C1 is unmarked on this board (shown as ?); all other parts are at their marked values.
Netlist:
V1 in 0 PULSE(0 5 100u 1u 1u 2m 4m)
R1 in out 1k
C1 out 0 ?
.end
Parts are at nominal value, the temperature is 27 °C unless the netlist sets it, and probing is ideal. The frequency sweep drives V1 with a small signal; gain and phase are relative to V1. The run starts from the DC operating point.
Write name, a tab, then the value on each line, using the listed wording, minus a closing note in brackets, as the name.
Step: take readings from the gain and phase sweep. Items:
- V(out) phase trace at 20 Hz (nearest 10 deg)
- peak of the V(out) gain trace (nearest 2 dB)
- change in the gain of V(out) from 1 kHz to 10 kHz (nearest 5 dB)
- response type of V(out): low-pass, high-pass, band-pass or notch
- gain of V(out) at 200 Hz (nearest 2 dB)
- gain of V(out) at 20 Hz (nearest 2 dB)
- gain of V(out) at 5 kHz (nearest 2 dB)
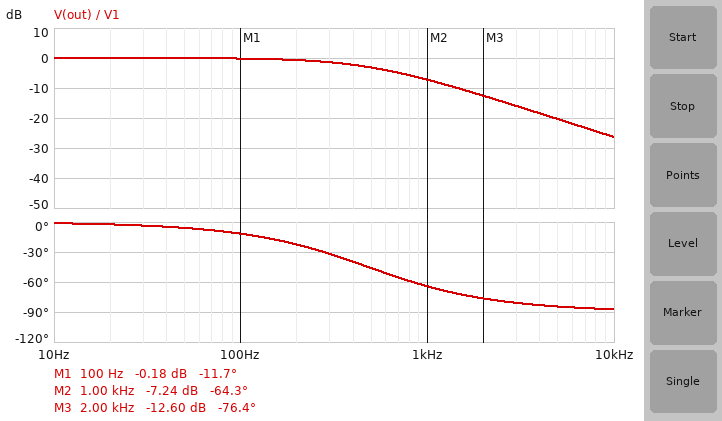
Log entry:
V(out) phase trace at 20 Hz	0 deg
peak of the V(out) gain trace	0 dB
change in the gain of V(out) from 1 kHz to 10 kHz	-20 dB
response type of V(out): low-pass, high-pass, band-pass or notch	low-pass
gain of V(out) at 200 Hz	0 dB
gain of V(out) at 20 Hz	0 dB
gain of V(out) at 5 kHz	-20 dB
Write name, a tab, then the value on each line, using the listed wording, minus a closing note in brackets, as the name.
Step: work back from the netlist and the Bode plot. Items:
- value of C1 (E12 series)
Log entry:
value of C1	330 nF
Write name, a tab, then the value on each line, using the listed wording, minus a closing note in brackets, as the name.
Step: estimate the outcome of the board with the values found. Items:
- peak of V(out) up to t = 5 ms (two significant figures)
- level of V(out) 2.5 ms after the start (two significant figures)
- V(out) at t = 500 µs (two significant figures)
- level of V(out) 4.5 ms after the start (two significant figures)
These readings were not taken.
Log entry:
peak of V(out) up to t = 5 ms	5.0 V
level of V(out) 2.5 ms after the start	1.5 V
V(out) at t = 500 µs	3.5 V
level of V(out) 4.5 ms after the start	3.5 V
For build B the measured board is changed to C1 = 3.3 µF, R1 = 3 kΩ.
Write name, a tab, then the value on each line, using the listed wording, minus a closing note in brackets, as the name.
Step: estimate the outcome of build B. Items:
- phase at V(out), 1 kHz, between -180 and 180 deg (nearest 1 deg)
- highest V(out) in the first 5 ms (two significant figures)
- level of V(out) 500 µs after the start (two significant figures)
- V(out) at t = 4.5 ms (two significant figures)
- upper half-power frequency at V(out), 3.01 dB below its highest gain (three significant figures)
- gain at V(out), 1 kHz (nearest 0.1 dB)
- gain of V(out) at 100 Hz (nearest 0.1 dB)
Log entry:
phase at V(out), 1 kHz, between -180 and 180 deg	-89 deg
highest V(out) in the first 5 ms	1.1 V
level of V(out) 500 µs after the start	200 mV
V(out) at t = 4.5 ms	920 mV
upper half-power frequency at V(out), 3.01 dB below its highest gain	16.1 Hz
gain at V(out), 1 kHz	-35.9 dB
gain of V(out) at 100 Hz	-16.0 dB
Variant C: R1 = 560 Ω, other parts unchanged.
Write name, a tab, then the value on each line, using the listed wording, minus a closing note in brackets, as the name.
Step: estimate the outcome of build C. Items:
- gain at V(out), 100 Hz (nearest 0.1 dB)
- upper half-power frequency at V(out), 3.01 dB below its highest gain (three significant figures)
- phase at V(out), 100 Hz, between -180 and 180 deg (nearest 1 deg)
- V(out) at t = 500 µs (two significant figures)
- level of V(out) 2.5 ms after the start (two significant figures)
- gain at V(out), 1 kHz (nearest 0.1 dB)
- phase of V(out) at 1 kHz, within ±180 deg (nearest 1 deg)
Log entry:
gain at V(out), 100 Hz	-0.1 dB
upper half-power frequency at V(out), 3.01 dB below its highest gain	861 Hz
phase at V(out), 100 Hz, between -180 and 180 deg	-7 deg
V(out) at t = 500 µs	4.4 V
level of V(out) 2.5 ms after the start	580 mV
gain at V(out), 1 kHz	-3.7 dB
phase of V(out) at 1 kHz, within ±180 deg	-49 deg
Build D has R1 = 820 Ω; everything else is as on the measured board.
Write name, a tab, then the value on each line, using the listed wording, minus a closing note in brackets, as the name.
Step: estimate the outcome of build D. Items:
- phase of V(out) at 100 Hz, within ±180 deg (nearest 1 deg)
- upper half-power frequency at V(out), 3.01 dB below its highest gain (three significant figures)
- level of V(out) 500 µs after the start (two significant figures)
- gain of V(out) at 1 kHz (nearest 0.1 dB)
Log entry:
phase of V(out) at 100 Hz, within ±180 deg	-10 deg
upper half-power frequency at V(out), 3.01 dB below its highest gain	588 Hz
level of V(out) 500 µs after the start	3.9 V
gain of V(out) at 1 kHz	-5.9 dB
